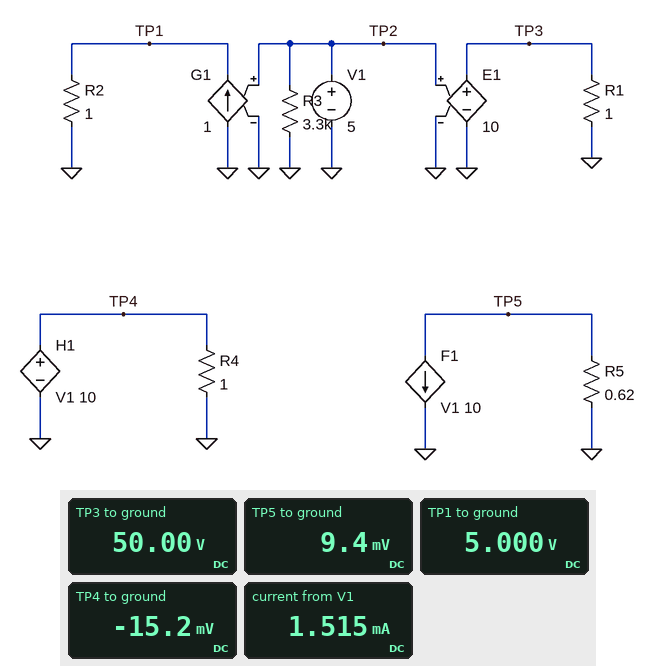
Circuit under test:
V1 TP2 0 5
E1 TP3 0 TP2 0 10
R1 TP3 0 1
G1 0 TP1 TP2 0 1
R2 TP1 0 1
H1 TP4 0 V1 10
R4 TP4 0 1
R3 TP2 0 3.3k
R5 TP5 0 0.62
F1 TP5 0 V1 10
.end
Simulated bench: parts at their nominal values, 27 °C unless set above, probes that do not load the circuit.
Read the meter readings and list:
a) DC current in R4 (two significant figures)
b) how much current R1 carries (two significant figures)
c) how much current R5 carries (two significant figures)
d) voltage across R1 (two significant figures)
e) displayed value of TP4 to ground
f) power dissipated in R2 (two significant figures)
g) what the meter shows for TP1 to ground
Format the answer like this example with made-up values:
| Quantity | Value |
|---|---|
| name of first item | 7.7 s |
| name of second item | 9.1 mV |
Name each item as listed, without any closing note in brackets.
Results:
| Quantity | Value |
|---|---|
| DC current in R4 | 15 mA |
| how much current R1 carries | 50 A |
| how much current R5 carries | 15 mA |
| voltage across R1 | 50 V |
| displayed value of TP4 to ground | -15.2 mV |
| power dissipated in R2 | 25 W |
| what the meter shows for TP1 to ground | 5.000 V |
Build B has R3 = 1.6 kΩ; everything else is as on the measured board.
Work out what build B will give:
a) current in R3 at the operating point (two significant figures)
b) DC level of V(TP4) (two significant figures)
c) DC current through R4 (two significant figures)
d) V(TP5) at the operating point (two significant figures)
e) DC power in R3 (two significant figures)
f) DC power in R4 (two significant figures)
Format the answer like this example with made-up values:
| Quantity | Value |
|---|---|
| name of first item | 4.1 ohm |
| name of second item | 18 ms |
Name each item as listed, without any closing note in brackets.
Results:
| Quantity | Value |
|---|---|
| current in R3 at the operating point | 3.1 mA |
| DC level of V(TP4) | -31 mV |
| DC current through R4 | 31 mA |
| V(TP5) at the operating point | 19 mV |
| DC power in R3 | 16 mW |
| DC power in R4 | 980 µW |
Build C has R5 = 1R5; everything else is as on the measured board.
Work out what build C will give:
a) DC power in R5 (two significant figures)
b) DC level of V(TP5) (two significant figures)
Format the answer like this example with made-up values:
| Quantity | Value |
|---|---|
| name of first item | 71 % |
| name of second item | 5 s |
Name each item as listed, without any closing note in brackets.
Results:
| Quantity | Value |
|---|---|
| DC power in R5 | 340 µW |
| DC level of V(TP5) | 23 mV |
